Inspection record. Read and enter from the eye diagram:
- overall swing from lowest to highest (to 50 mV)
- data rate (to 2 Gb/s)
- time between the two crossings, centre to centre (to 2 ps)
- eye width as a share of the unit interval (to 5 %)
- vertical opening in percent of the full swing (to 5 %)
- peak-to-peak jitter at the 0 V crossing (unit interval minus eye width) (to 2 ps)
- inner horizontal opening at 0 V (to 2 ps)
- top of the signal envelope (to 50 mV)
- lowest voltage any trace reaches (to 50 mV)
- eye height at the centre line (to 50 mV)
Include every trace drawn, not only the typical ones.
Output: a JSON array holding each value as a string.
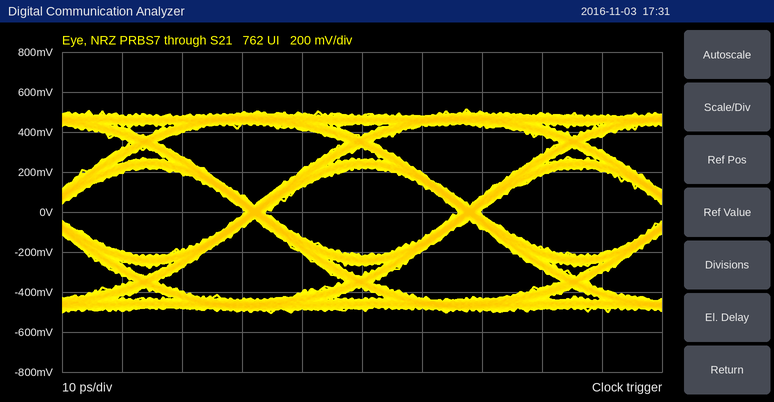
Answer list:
["1.00 V", "28 Gb/s", "36 ps", "90 %", "45 %", "4 ps", "32 ps", "500 mV", "-500 mV", "450 mV"]
